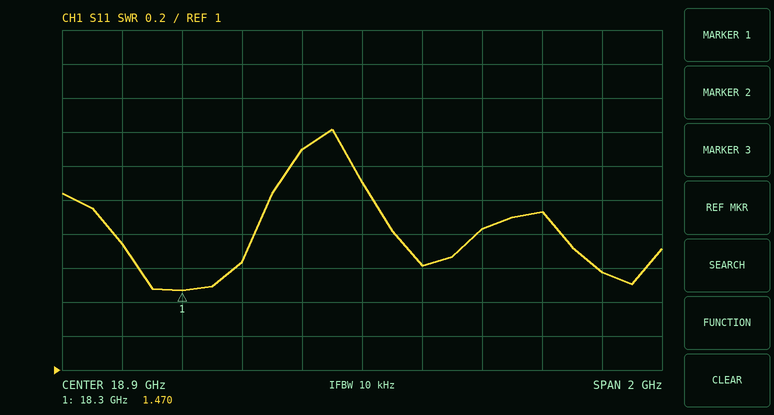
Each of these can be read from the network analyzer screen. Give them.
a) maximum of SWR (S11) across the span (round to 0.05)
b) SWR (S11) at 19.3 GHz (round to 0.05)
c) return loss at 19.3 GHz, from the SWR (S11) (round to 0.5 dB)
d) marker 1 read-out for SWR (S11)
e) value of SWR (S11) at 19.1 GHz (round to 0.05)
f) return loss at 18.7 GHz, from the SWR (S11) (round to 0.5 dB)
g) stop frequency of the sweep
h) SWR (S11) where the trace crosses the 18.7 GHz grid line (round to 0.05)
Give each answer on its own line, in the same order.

2.40
1.85
10.5 dB
1.470
1.60
8.0 dB
19.9 GHz
2.30
